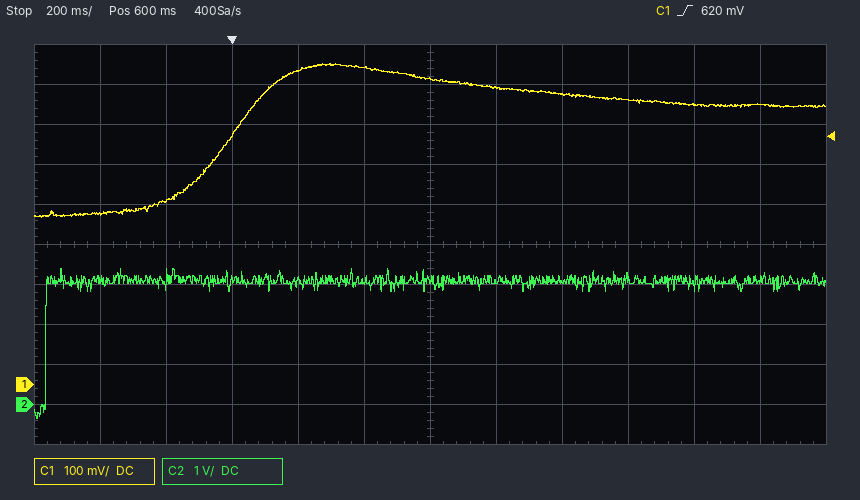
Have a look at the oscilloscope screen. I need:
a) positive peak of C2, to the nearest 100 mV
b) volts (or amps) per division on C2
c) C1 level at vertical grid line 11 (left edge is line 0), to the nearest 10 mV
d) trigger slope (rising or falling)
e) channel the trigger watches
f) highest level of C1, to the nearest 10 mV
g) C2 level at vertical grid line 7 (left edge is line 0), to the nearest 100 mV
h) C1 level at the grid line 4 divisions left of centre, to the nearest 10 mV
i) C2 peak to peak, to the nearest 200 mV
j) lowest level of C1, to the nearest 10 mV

3.4 V
1 V
700 mV
rising
C1
800 mV
3.1 V
460 mV
3.8 V
420 mV
